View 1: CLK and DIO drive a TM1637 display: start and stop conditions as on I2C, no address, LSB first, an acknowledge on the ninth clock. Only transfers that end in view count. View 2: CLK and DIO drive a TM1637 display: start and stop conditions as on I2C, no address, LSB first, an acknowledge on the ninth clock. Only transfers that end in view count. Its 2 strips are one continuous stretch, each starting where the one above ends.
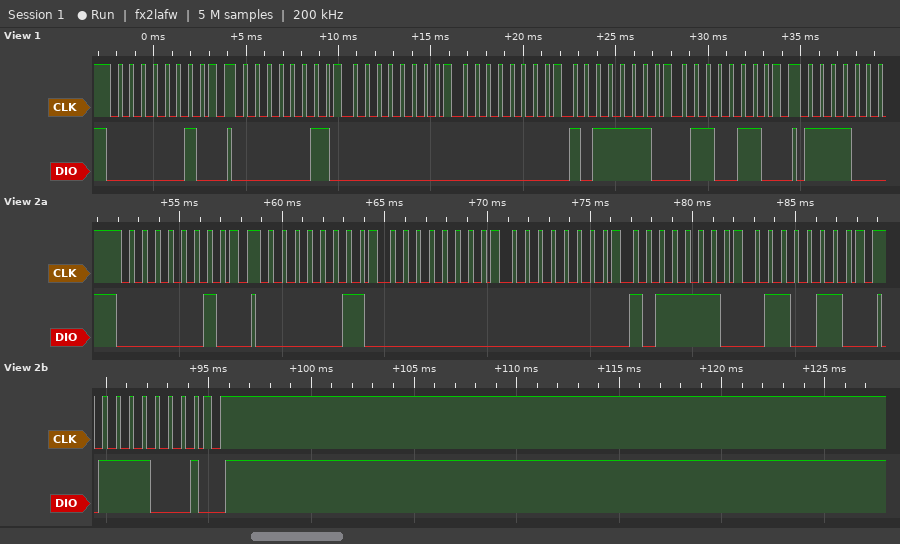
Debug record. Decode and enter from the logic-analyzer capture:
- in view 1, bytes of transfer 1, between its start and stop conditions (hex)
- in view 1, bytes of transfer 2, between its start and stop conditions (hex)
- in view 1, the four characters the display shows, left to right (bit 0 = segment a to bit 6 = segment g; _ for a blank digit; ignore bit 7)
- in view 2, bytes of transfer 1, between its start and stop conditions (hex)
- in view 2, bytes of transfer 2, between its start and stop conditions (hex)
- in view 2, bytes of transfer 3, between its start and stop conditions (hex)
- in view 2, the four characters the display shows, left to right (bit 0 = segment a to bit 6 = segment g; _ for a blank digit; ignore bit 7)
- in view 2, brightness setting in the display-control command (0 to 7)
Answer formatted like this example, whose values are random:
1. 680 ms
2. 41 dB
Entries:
1. 40
2. C0 00 00 7D 66
3. __64
4. 40
5. C0 00 00 7D 66
6. 8F
7. __64
8. 7
